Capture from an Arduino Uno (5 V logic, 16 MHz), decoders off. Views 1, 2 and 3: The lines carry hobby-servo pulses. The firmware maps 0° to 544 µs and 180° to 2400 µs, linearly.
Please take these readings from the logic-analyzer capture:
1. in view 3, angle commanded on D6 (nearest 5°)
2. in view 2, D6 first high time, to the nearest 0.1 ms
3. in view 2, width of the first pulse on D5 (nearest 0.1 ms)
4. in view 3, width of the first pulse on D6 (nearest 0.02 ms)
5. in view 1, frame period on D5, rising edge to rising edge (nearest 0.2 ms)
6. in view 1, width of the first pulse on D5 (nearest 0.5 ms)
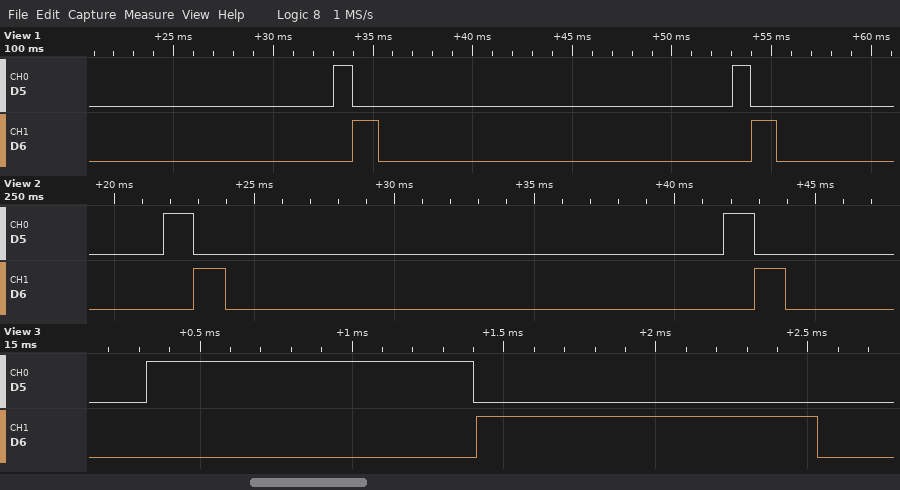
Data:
55°
1.1 ms
1.1 ms
1.12 ms
20.0 ms
1.0 ms
